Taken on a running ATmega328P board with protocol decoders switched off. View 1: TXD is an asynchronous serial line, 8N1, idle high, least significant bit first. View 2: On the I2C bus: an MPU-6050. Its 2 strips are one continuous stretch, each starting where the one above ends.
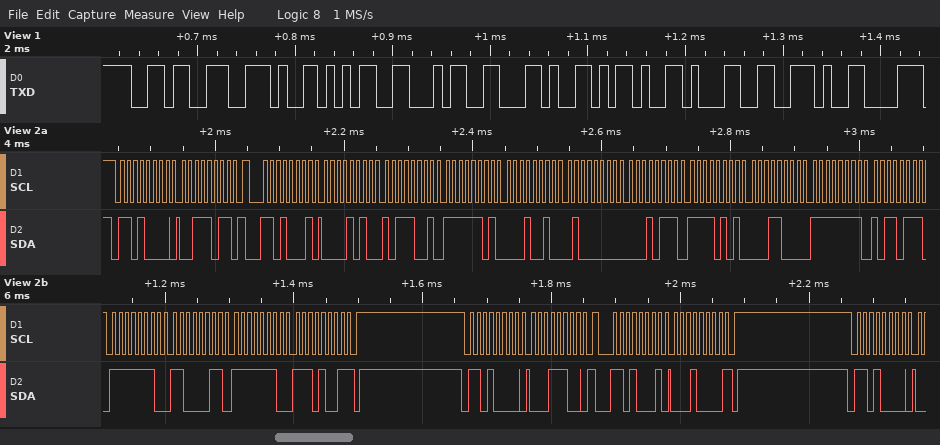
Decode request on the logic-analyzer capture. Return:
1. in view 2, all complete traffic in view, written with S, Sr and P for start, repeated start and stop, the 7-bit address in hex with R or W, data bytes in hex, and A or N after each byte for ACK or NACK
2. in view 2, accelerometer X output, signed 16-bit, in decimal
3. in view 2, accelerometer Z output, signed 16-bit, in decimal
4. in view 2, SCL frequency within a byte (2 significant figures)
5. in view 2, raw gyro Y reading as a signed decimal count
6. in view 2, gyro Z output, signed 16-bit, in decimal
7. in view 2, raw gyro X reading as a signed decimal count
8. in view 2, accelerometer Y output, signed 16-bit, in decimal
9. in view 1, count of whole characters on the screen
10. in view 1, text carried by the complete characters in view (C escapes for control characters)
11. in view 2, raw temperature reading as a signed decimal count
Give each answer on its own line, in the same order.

S 68W A 3B A Sr 68R A 0A A B9 A FD A 12 A 40 A 17 A F5 A 18 A FF A B7 A FE A C3 A FE A E9 N P S 68W A 1C A Sr 68R A 10 N P S 68W A
2745
16407
100 kHz
-317
-279
-73
-750
8
"6.54,-1."
-2792
